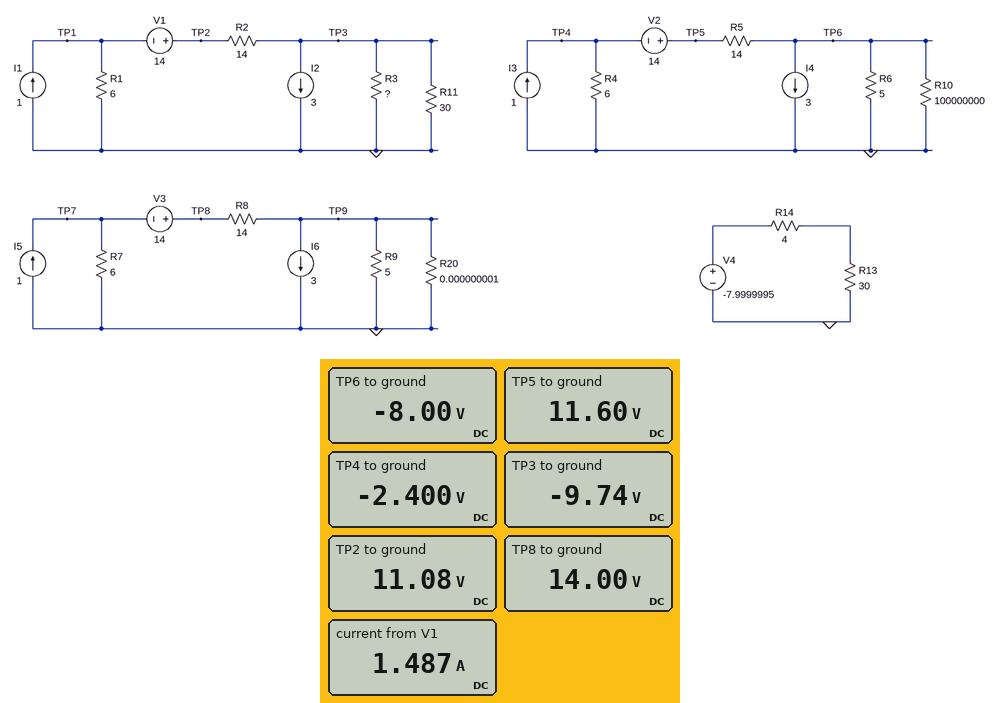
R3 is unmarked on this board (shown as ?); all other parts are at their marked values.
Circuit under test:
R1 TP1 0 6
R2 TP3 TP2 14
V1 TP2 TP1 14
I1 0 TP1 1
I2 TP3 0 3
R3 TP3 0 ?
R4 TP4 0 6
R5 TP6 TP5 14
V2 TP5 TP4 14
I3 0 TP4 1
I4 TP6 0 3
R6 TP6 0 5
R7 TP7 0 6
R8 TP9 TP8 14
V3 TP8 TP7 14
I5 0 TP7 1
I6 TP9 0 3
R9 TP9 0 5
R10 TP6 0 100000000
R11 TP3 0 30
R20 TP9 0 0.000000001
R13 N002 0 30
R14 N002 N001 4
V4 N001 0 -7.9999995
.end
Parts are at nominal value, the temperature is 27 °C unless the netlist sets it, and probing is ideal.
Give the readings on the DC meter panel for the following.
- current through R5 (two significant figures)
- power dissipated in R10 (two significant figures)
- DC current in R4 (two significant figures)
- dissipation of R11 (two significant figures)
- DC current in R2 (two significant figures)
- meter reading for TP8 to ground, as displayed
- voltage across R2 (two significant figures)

1.4 A
640 nW
400 mA
3.2 W
1.5 A
14.00 V
21 V
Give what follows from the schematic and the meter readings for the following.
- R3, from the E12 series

8.2 Ω
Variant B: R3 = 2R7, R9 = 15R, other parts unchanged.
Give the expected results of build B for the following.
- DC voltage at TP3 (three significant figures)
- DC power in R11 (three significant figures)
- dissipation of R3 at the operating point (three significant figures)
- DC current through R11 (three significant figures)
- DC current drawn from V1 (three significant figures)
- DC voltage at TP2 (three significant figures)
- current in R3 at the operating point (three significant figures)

-4.41 V
648 mW
7.20 W
147 mA
1.22 A
12.7 V
1.63 A
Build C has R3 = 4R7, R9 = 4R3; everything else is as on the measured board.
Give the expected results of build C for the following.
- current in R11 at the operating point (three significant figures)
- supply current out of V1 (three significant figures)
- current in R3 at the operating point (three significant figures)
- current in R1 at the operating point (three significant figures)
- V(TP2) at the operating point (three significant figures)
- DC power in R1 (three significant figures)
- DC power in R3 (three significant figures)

225 mA
1.34 A
1.44 A
338 mA
12.0 V
684 mW
9.71 W
